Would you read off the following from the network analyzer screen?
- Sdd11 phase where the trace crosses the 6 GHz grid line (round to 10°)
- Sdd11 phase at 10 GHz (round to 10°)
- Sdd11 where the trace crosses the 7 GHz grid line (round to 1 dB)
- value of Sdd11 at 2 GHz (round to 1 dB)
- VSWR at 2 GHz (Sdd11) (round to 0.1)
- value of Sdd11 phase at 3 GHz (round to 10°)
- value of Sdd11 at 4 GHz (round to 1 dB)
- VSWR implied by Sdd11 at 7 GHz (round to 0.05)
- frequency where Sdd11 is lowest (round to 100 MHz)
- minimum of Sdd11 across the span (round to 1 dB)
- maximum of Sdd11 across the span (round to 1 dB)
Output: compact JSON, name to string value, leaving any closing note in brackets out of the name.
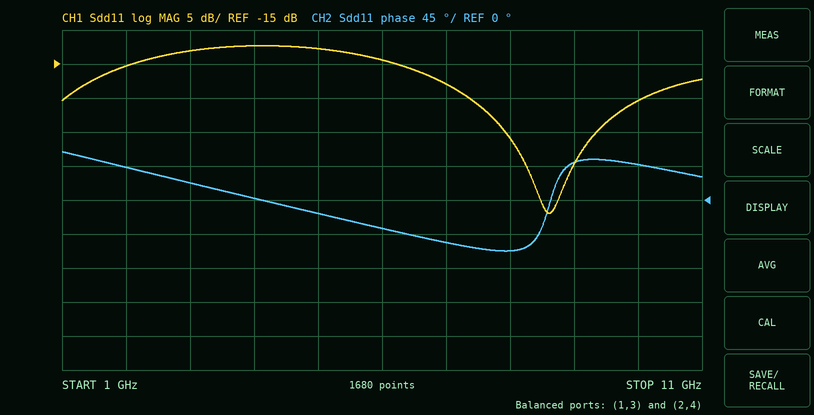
{"Sdd11 phase where the trace crosses the 6 GHz grid line": "-40°", "Sdd11 phase at 10 GHz": "50°", "Sdd11 where the trace crosses the 7 GHz grid line": "-18 dB", "value of Sdd11 at 2 GHz": "-15 dB", "VSWR at 2 GHz (Sdd11)": "1.4", "value of Sdd11 phase at 3 GHz": "20°", "value of Sdd11 at 4 GHz": "-12 dB", "VSWR implied by Sdd11 at 7 GHz": "1.30", "frequency where Sdd11 is lowest": "8.6 GHz", "minimum of Sdd11 across the span": "-37 dB", "maximum of Sdd11 across the span": "-12 dB"}
